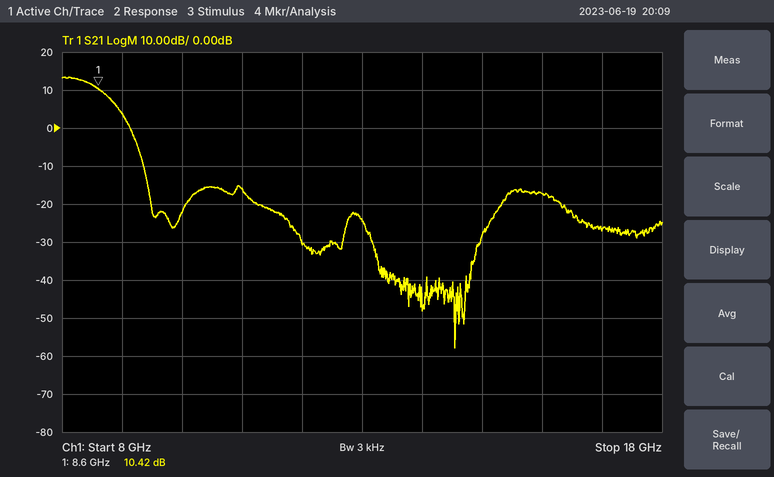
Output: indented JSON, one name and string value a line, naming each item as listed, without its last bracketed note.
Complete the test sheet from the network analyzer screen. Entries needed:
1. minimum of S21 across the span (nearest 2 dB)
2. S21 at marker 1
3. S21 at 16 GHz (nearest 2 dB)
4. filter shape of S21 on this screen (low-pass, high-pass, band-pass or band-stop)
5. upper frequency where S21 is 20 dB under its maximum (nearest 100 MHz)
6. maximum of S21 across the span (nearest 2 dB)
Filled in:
{
  "minimum of S21 across the span": "-58 dB",
  "S21 at marker 1": "10.42 dB",
  "S21 at 16 GHz": "-18 dB",
  "filter shape of S21 on this screen": "low-pass",
  "upper frequency where S21 is 20 dB under its maximum": "9.3 GHz",
  "maximum of S21 across the span": "14 dB"
}
